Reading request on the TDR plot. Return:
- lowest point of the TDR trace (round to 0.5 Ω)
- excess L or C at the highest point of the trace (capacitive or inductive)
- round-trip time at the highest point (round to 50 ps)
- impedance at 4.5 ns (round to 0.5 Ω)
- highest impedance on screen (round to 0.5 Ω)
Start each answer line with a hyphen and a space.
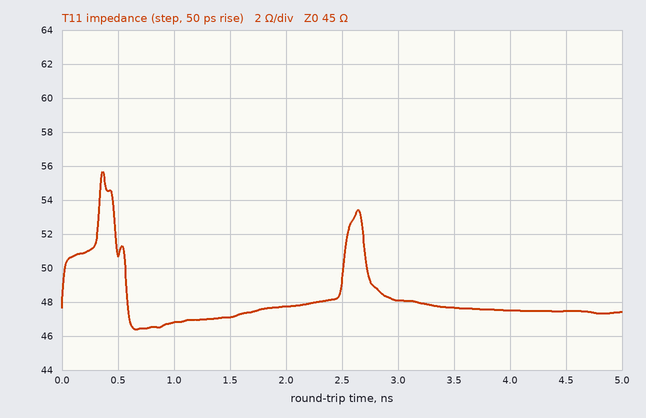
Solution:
- 46.5 Ω
- inductive
- 350 ps
- 47.5 Ω
- 55.5 Ω
